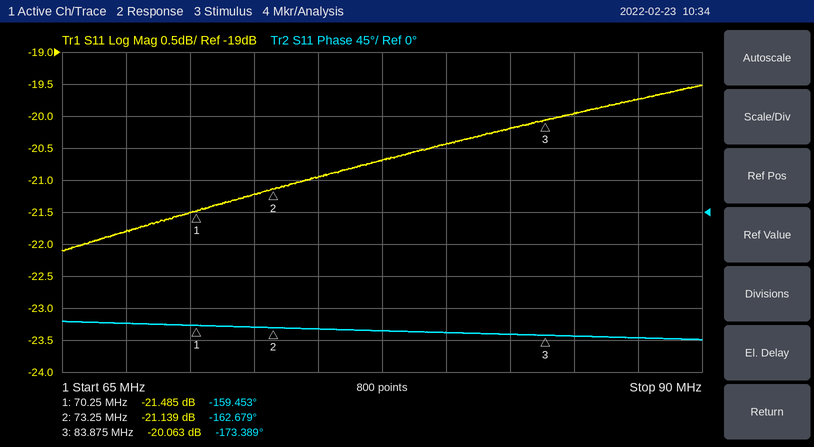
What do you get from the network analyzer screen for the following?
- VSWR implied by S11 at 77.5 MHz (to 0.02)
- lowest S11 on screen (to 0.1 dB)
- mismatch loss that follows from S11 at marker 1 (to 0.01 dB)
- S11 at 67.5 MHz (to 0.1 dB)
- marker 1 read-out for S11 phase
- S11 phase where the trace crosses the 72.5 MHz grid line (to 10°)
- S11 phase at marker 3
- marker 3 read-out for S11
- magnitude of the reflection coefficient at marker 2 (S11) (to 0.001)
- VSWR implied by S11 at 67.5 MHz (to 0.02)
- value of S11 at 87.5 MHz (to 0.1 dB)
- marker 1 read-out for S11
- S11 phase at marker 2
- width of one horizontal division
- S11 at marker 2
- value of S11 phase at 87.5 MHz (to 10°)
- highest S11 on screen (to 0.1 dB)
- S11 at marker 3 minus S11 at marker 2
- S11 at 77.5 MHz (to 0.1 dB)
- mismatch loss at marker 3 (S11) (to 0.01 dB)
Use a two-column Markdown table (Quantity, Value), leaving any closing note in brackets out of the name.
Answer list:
| Quantity | Value |
|---|---|
| VSWR implied by S11 at 77.5 MHz | 1.20 |
| lowest S11 on screen | -22.1 dB |
| mismatch loss that follows from S11 at marker 1 | 0.03 dB |
| S11 at 67.5 MHz | -21.8 dB |
| marker 1 read-out for S11 phase | -159.453° |
| S11 phase where the trace crosses the 72.5 MHz grid line | -160° |
| S11 phase at marker 3 | -173.389° |
| marker 3 read-out for S11 | -20.063 dB |
| magnitude of the reflection coefficient at marker 2 (S11) | 0.088 |
| VSWR implied by S11 at 67.5 MHz | 1.18 |
| value of S11 at 87.5 MHz | -19.7 dB |
| marker 1 read-out for S11 | -21.485 dB |
| S11 phase at marker 2 | -162.679° |
| width of one horizontal division | 2.5 MHz |
| S11 at marker 2 | -21.139 dB |
| value of S11 phase at 87.5 MHz | -180° |
| highest S11 on screen | -19.5 dB |
| S11 at marker 3 minus S11 at marker 2 | 1.076 dB |
| S11 at 77.5 MHz | -20.7 dB |
| mismatch loss at marker 3 (S11) | 0.04 dB |
